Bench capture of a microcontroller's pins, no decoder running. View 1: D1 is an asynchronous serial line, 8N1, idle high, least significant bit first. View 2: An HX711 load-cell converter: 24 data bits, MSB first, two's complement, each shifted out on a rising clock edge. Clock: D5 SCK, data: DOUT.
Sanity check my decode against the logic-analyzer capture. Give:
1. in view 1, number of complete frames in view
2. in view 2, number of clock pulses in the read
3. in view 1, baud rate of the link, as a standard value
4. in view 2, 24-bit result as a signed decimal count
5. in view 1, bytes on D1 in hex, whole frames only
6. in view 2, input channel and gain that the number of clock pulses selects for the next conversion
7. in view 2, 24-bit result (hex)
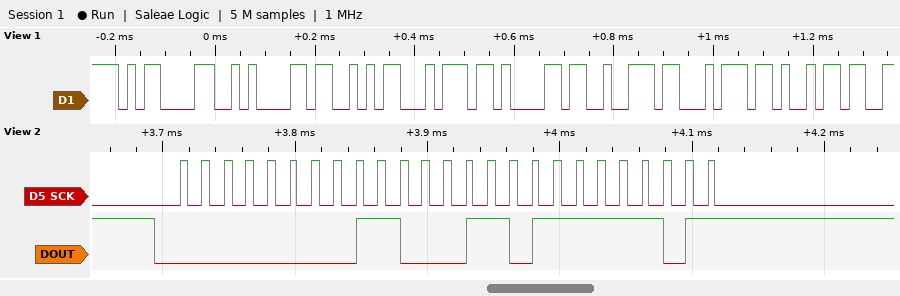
8
25
57600 baud
50941
0D 0A 53 74 61 72 74 69
channel A, gain 128
0x00C6FD
